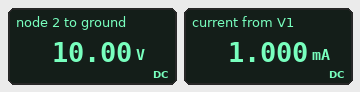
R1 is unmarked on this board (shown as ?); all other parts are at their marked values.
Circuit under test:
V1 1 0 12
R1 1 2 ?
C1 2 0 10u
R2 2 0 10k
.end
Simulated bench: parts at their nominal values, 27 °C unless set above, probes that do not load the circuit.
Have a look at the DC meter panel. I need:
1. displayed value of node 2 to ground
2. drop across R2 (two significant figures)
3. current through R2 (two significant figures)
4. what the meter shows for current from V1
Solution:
10.00 V
10 V
1.0 mA
1.000 mA
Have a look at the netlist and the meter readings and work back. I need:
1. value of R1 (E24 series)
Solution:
2 kΩ
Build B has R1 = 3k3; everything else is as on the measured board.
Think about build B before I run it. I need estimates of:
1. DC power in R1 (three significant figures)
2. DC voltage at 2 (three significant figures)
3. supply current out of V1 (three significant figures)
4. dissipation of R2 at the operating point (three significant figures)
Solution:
2.69 mW
9.02 V
902 µA
8.14 mW
